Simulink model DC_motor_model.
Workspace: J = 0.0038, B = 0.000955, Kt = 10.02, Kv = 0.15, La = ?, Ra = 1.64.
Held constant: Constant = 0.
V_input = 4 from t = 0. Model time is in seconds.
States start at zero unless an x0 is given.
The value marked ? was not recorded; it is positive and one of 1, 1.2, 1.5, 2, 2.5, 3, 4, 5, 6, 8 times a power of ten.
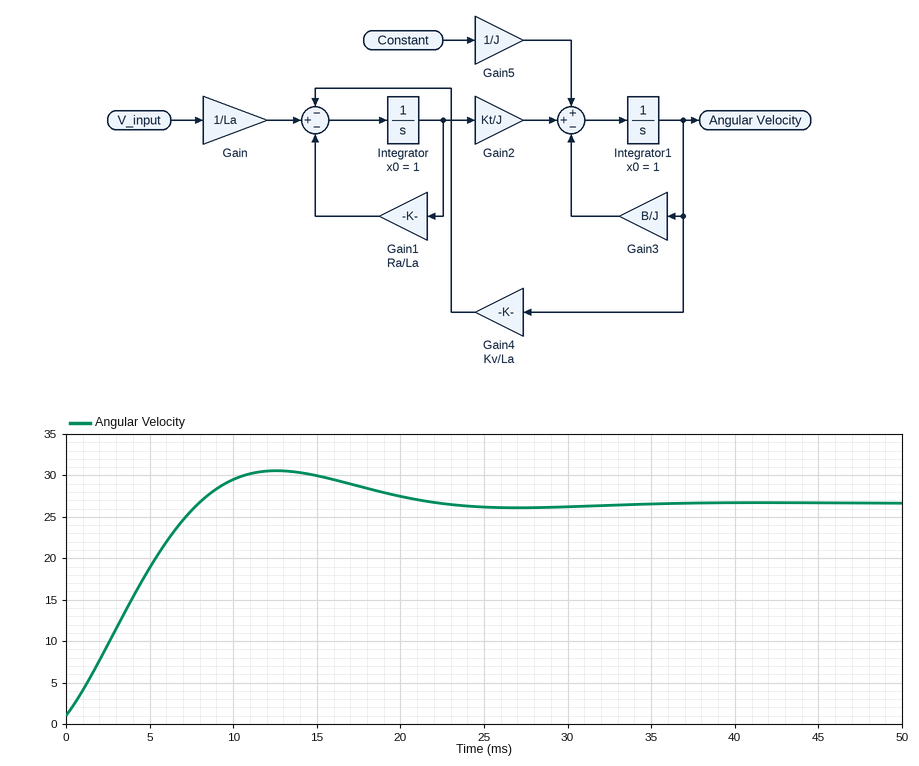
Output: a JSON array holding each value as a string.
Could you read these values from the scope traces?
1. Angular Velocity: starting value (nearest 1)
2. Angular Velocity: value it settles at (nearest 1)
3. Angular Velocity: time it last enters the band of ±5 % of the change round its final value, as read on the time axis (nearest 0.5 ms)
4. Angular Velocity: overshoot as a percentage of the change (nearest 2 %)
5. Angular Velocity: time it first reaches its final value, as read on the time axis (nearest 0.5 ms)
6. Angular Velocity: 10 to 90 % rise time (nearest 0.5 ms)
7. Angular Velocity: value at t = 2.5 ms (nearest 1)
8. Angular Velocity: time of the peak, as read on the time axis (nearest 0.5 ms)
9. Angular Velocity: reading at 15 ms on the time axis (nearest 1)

["1", "27", "19.0 ms", "16 %", "8.0 ms", "6.0 ms", "10", "12.5 ms", "30"]
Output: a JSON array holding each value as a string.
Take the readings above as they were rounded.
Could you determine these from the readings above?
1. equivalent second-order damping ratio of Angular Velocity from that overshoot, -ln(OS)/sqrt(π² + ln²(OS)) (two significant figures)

["0.50"]
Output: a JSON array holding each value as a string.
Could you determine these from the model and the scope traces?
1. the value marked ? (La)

["0.006"]
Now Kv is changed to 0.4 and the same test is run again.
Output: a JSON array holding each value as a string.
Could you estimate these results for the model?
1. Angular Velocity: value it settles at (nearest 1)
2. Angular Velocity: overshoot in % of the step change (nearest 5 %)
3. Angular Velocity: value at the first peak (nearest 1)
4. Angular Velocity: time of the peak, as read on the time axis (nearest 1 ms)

["10", "45 %", "14", "6 ms"]
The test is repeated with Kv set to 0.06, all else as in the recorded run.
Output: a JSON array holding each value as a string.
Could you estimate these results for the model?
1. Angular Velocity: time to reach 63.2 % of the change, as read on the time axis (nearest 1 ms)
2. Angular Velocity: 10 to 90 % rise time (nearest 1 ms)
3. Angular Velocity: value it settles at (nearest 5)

["10 ms", "16 ms", "65"]
